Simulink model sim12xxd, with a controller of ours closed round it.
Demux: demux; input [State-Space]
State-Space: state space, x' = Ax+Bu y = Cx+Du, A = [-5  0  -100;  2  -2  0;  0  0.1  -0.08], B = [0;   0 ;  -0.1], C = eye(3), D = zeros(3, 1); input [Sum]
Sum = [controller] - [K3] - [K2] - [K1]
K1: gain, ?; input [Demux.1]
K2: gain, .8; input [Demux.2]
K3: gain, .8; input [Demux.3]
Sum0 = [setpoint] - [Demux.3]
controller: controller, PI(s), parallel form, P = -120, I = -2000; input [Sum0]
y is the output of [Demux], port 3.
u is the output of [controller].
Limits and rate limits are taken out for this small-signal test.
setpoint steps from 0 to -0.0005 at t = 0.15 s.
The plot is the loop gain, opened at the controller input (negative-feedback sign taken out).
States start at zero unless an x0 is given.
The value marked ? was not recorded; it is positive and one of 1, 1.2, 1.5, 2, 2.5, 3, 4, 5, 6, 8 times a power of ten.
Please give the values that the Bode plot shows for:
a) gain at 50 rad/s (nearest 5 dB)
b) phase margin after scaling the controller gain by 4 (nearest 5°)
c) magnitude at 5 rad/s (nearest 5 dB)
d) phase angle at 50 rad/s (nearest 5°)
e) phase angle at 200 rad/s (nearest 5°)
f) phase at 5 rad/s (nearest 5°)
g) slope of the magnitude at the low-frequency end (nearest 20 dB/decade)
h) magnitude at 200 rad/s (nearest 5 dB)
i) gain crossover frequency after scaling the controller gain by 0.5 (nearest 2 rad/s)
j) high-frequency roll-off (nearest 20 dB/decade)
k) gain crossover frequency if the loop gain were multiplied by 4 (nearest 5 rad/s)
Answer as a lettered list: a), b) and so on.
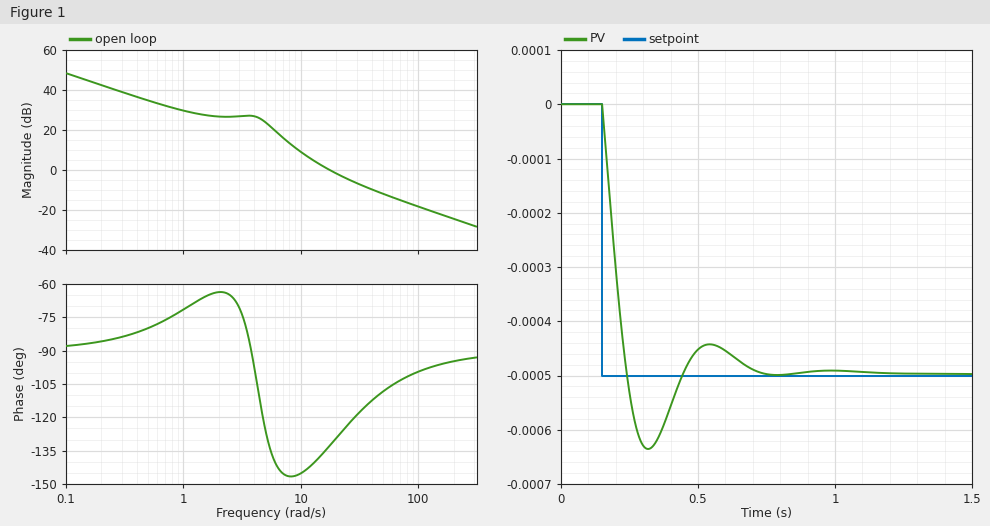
a) -10 dB
b) 70°
c) 25 dB
d) -110°
e) -95°
f) -125°
g) -20 dB/decade
h) -25 dB
i) 12 rad/s
j) -20 dB/decade
k) 50 rad/s
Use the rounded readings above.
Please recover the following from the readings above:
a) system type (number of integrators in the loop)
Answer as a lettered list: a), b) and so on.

a) 1
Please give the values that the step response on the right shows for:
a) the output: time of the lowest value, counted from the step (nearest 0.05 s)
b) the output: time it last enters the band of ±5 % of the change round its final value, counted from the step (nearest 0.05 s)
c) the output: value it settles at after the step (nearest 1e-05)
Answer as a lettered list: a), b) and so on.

a) 0.15 s
b) 0.50 s
c) -0.00050
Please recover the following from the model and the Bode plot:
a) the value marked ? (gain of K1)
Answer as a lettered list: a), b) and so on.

a) 2
